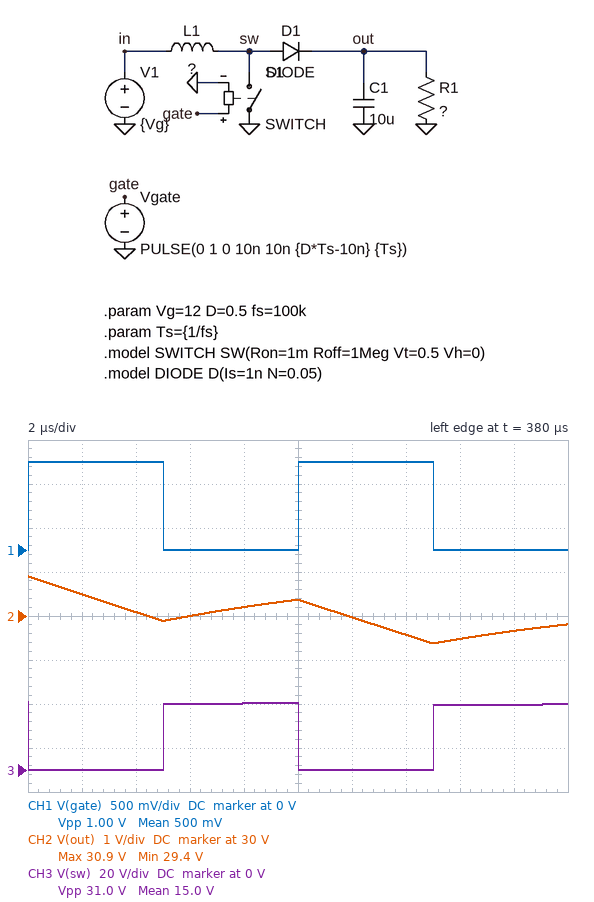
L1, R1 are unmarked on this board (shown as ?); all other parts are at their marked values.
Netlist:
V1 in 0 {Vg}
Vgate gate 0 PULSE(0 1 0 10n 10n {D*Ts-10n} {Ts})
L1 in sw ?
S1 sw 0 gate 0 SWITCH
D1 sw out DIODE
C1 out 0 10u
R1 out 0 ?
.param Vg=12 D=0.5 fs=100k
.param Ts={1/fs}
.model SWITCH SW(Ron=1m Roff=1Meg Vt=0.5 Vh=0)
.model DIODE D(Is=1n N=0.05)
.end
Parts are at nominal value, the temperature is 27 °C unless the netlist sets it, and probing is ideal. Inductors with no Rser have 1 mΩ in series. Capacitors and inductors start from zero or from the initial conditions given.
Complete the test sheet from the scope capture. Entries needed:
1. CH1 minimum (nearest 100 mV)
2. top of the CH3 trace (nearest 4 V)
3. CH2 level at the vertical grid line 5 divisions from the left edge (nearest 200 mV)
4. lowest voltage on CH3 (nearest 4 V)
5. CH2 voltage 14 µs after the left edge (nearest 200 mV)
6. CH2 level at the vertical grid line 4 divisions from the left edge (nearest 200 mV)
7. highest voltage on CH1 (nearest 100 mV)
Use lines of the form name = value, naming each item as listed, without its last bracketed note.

CH1 minimum = 0 V
top of the CH3 trace = 32 V
CH2 level at the vertical grid line 5 divisions from the left edge = 30.4 V
lowest voltage on CH3 = 0 V
CH2 voltage 14 µs after the left edge = 29.6 V
CH2 level at the vertical grid line 4 divisions from the left edge = 30.2 V
highest voltage on CH1 = 1.0 V
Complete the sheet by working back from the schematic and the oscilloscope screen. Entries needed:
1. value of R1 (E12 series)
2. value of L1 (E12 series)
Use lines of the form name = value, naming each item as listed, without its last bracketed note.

value of R1 = 15 Ω
value of L1 = 220 µH
